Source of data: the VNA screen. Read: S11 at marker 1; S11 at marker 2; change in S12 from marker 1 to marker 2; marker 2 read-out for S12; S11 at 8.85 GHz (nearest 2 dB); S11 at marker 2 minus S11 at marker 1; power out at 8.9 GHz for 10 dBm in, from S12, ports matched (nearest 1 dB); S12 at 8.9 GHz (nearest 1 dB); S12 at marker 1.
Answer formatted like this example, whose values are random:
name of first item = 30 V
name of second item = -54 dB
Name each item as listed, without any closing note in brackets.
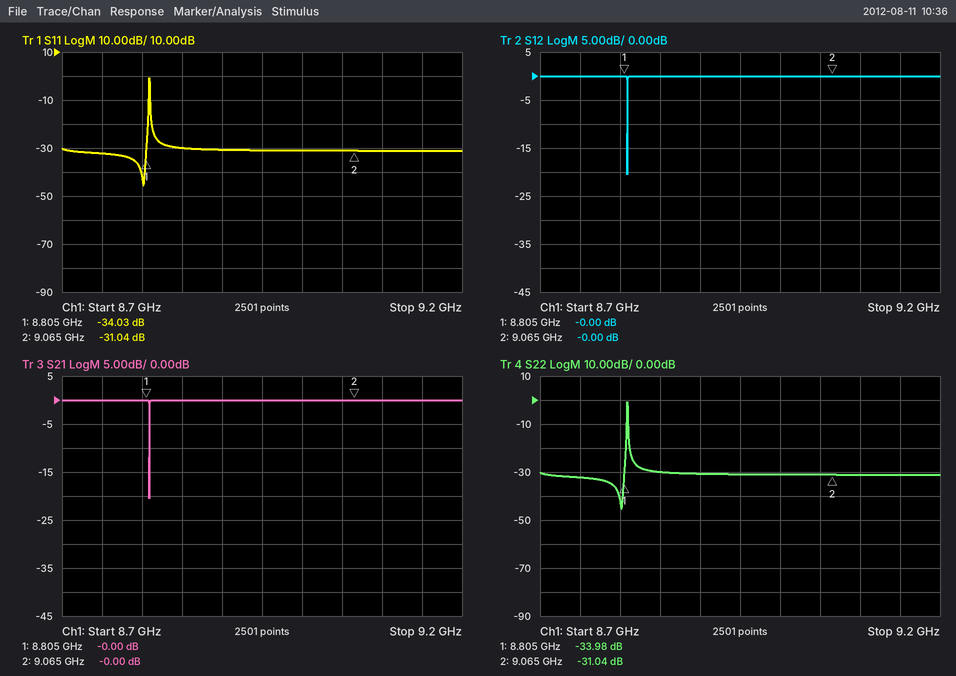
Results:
S11 at marker 1 = -34.03 dB
S11 at marker 2 = -31.04 dB
change in S12 from marker 1 to marker 2 = 0.00 dB
marker 2 read-out for S12 = -0.00 dB
S11 at 8.85 GHz = -30 dB
S11 at marker 2 minus S11 at marker 1 = 2.99 dB
power out at 8.9 GHz for 10 dBm in, from S12, ports matched = 10 dBm
S12 at 8.9 GHz = 0 dB
S12 at marker 1 = -0.00 dB
